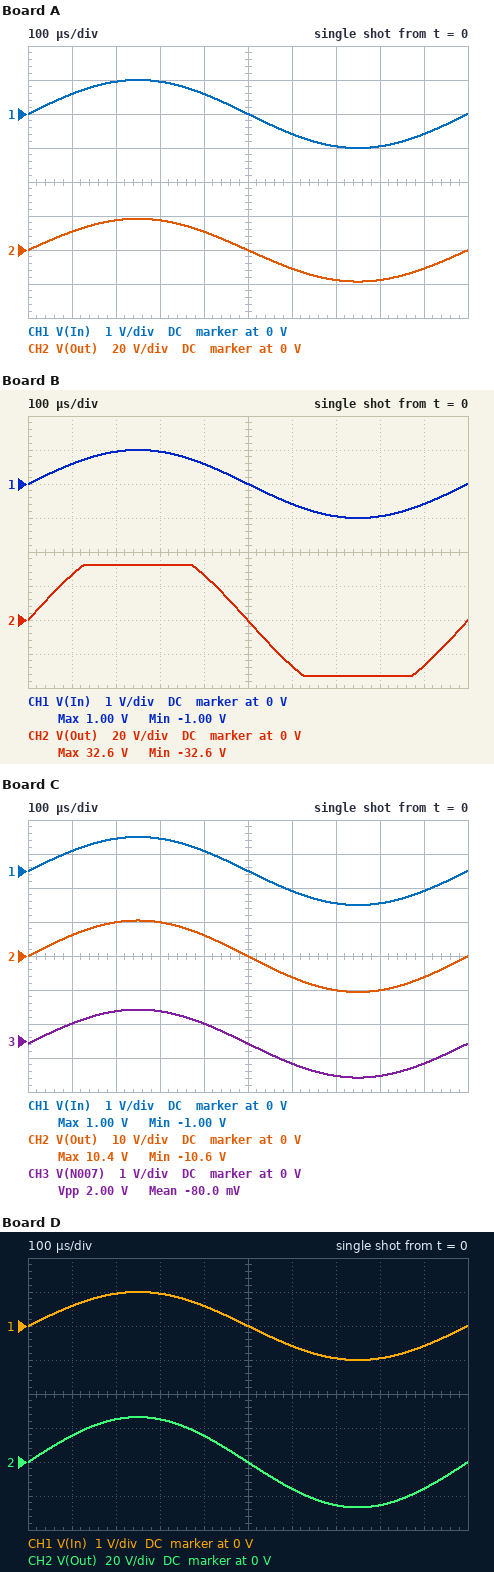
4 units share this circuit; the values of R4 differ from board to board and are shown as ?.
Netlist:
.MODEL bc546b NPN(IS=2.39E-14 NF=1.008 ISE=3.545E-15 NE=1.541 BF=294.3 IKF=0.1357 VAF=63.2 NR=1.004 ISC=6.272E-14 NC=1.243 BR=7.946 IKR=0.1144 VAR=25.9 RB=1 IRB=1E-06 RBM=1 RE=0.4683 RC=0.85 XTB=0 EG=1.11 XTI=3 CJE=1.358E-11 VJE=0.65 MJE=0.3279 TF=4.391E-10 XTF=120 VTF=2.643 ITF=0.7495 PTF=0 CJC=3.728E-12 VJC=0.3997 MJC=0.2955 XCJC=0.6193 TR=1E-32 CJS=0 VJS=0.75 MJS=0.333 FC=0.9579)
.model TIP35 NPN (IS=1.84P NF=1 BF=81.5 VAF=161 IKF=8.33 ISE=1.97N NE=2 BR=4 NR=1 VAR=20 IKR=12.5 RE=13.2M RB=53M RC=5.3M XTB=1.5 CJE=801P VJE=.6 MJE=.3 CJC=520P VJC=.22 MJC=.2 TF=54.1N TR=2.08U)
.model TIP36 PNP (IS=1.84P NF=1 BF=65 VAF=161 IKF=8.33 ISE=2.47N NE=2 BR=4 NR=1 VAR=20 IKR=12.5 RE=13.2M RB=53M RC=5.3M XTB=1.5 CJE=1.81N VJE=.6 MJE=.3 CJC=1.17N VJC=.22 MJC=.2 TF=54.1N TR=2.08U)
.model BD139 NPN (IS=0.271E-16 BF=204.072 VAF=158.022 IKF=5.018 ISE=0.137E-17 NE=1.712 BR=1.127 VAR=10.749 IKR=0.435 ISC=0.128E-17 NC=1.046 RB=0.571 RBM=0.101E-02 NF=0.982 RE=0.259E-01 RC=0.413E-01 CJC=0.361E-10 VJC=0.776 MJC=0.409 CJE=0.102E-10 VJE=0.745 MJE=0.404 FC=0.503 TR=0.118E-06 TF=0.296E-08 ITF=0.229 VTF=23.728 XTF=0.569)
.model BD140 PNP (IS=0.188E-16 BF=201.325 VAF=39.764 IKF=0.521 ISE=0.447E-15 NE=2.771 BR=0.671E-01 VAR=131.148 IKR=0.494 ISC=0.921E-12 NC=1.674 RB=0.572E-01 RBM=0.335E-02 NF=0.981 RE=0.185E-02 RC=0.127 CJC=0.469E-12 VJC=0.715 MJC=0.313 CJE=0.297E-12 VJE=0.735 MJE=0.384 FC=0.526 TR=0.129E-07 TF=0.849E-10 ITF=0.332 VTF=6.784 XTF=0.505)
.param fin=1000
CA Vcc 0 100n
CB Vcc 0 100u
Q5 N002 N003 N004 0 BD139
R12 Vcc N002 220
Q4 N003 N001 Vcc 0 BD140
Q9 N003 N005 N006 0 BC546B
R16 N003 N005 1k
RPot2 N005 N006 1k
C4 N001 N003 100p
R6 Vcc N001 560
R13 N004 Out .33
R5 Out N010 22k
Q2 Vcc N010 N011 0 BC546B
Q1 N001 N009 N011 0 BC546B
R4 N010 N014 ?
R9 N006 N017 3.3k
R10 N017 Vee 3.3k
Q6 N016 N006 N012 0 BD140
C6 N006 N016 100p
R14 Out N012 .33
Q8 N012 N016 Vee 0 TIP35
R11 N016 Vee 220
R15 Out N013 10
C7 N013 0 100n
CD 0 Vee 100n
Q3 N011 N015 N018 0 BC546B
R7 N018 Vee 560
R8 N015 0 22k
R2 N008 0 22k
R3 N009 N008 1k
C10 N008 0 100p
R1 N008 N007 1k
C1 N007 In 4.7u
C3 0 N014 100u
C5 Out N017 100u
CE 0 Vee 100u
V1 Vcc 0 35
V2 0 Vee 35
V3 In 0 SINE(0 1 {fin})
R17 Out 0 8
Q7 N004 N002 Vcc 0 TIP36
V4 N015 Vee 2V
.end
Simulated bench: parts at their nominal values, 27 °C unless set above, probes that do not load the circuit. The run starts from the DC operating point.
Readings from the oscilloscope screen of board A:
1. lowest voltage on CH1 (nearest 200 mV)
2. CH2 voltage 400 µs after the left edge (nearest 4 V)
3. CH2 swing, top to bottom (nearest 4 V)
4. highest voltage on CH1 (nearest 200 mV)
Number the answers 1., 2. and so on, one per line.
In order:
1. -1.0 V
2. 12 V
3. 36 V
4. 1.0 V
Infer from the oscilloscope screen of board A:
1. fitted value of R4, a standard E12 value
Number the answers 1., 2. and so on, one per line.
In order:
1. 1.2 kΩ
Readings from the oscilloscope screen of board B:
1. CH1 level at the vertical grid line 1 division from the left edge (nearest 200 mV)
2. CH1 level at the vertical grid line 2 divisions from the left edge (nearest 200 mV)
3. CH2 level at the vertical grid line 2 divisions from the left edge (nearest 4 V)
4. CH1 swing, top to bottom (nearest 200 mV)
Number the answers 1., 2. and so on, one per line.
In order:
1. 600 mV
2. 1.0 V
3. 32 V
4. 2.0 V
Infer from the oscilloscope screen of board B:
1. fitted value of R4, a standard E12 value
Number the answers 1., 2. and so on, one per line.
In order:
1. 470 Ω
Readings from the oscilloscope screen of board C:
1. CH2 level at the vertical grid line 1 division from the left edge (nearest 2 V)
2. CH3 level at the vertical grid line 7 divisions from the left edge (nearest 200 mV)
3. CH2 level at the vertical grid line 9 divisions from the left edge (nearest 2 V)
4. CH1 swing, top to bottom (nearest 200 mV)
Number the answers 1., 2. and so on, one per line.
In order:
1. 6 V
2. -1.0 V
3. -6 V
4. 2.0 V
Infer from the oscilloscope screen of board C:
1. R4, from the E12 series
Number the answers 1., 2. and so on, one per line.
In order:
1. 2.2 kΩ
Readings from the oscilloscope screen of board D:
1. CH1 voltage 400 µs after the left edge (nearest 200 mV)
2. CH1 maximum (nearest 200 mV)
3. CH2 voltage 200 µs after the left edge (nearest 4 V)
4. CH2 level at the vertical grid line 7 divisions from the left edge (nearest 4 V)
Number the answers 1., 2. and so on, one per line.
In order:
1. 600 mV
2. 1.0 V
3. 24 V
4. -24 V
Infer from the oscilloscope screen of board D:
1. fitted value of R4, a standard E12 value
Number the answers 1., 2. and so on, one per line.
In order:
1. 820 Ω
